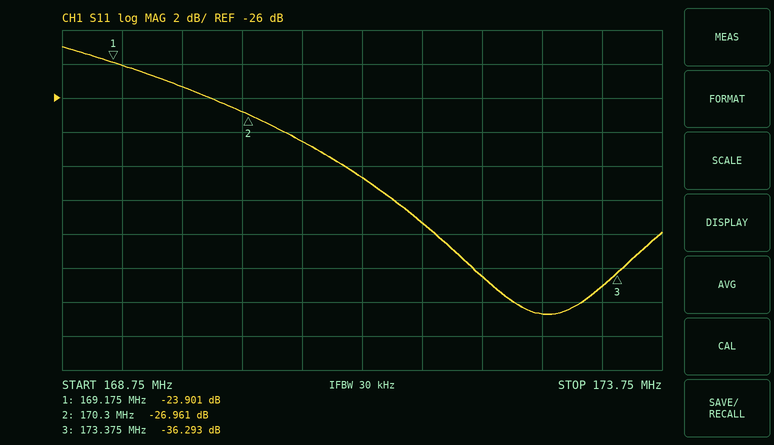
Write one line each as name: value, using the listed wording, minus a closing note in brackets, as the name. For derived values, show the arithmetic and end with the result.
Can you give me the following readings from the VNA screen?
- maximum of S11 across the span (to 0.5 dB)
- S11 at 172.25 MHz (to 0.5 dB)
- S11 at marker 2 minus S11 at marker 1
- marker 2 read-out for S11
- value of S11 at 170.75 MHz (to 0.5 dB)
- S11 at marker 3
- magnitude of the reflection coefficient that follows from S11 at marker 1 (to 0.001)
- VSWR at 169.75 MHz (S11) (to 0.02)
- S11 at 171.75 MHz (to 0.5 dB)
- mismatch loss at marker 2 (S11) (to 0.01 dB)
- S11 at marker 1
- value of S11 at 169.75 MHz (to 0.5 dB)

maximum of S11 across the span: -23.0 dB
S11 at 172.25 MHz: -36.5 dB
S11 at marker 2 minus S11 at marker 1: -26.961 − (-23.901) = -3.060 dB
marker 2 read-out for S11: -26.961 dB
value of S11 at 170.75 MHz: -28.5 dB
S11 at marker 3: -36.293 dB
magnitude of the reflection coefficient that follows from S11 at marker 1: 10^(-23.901/20) ≈ 0.064
VSWR at 169.75 MHz (S11): |Γ| = 10^(-25.5/20) = 0.0531; VSWR = (1 + 0.0531)/(1 − 0.0531) ≈ 1.11, so 1.12 to the nearest 0.02
S11 at 171.75 MHz: -33.5 dB
mismatch loss at marker 2 (S11): −10 log10(1 − 10^(-26.961/10)) ≈ 0.01 dB
S11 at marker 1: -23.901 dB
value of S11 at 169.75 MHz: -25.5 dB
